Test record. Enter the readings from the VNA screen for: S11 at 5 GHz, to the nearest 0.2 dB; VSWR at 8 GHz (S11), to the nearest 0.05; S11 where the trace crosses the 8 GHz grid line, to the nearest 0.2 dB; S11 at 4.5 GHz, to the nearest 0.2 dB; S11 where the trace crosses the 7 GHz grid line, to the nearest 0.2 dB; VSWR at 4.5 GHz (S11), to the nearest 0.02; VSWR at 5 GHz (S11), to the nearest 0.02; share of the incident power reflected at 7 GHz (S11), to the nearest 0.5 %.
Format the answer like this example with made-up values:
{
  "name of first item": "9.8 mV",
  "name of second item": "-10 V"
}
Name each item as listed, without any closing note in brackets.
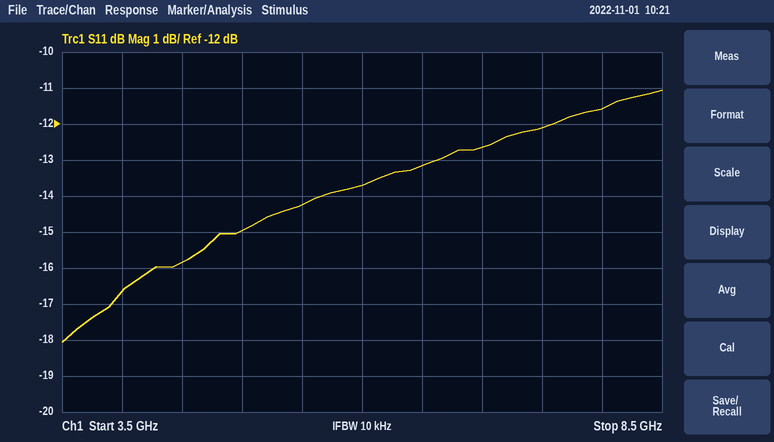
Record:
{
  "S11 at 5 GHz, to the nearest 0.2 dB": "-15.0 dB",
  "VSWR at 8 GHz (S11), to the nearest 0.05": "1.70",
  "S11 where the trace crosses the 8 GHz grid line, to the nearest 0.2 dB": "-11.6 dB",
  "S11 at 4.5 GHz, to the nearest 0.2 dB": "-15.8 dB",
  "S11 where the trace crosses the 7 GHz grid line, to the nearest 0.2 dB": "-12.6 dB",
  "VSWR at 4.5 GHz (S11), to the nearest 0.02": "1.38",
  "VSWR at 5 GHz (S11), to the nearest 0.02": "1.44",
  "share of the incident power reflected at 7 GHz (S11), to the nearest 0.5 %": "5.5 %"
}
